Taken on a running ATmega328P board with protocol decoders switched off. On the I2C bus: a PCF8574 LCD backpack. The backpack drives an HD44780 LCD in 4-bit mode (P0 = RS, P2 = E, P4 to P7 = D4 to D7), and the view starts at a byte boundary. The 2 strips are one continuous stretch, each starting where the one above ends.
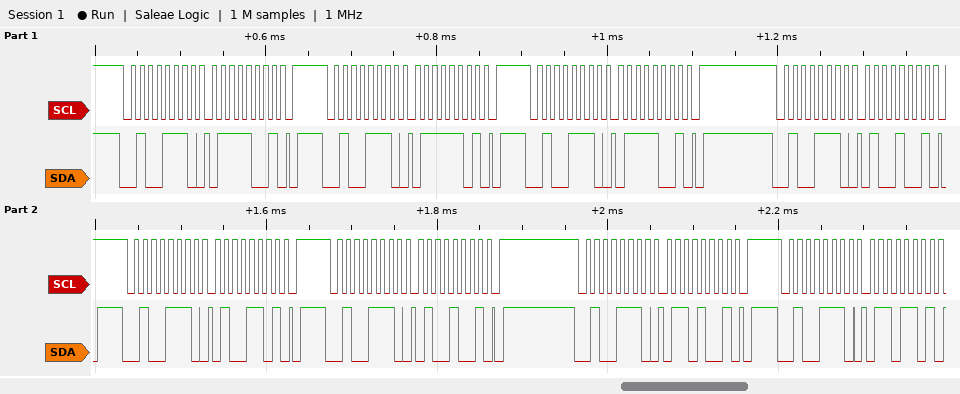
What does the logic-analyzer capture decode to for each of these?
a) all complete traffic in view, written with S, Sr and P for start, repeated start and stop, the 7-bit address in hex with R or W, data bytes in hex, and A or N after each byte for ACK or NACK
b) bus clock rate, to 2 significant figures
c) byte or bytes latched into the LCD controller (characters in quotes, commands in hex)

S 27W A 79 A P S 27W A 7D A P S 27W A 79 A P S 27W A 49 A P S 27W A 4D A P S 27W A 49 A P S 27W A 69 A P S 27W A 6D A
100 kHz
't'
